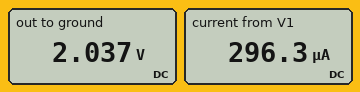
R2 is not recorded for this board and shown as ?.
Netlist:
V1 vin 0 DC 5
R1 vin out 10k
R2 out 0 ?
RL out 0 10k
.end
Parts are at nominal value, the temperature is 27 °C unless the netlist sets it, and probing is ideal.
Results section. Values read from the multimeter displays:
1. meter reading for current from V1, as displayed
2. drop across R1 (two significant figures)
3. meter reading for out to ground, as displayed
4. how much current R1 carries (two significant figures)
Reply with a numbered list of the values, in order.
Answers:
1. 296.3 µA
2. 3.0 V
3. 2.037 V
4. 300 µA
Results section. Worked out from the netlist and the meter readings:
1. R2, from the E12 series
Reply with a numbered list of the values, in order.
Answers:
1. 22 kΩ
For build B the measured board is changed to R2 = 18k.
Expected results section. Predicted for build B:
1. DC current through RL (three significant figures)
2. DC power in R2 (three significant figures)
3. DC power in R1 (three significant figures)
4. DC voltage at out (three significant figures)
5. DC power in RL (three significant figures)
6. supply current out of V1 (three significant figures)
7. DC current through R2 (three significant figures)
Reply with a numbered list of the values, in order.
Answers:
1. 196 µA
2. 213 µW
3. 926 µW
4. 1.96 V
5. 383 µW
6. 304 µA
7. 109 µA
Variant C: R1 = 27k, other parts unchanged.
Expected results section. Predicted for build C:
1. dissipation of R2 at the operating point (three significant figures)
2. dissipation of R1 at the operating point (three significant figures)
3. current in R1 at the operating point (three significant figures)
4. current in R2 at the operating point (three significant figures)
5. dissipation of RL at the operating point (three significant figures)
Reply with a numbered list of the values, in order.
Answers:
1. 46.8 µW
2. 588 µW
3. 148 µA
4. 46.1 µA
5. 103 µW
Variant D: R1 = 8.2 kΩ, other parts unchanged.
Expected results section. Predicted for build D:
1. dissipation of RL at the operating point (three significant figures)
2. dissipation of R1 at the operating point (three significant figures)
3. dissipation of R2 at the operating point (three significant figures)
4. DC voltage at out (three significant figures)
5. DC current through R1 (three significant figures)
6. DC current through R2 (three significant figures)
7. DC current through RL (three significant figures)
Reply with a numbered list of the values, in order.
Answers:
1. 520 µW
2. 902 µW
3. 236 µW
4. 2.28 V
5. 332 µA
6. 104 µA
7. 228 µA
